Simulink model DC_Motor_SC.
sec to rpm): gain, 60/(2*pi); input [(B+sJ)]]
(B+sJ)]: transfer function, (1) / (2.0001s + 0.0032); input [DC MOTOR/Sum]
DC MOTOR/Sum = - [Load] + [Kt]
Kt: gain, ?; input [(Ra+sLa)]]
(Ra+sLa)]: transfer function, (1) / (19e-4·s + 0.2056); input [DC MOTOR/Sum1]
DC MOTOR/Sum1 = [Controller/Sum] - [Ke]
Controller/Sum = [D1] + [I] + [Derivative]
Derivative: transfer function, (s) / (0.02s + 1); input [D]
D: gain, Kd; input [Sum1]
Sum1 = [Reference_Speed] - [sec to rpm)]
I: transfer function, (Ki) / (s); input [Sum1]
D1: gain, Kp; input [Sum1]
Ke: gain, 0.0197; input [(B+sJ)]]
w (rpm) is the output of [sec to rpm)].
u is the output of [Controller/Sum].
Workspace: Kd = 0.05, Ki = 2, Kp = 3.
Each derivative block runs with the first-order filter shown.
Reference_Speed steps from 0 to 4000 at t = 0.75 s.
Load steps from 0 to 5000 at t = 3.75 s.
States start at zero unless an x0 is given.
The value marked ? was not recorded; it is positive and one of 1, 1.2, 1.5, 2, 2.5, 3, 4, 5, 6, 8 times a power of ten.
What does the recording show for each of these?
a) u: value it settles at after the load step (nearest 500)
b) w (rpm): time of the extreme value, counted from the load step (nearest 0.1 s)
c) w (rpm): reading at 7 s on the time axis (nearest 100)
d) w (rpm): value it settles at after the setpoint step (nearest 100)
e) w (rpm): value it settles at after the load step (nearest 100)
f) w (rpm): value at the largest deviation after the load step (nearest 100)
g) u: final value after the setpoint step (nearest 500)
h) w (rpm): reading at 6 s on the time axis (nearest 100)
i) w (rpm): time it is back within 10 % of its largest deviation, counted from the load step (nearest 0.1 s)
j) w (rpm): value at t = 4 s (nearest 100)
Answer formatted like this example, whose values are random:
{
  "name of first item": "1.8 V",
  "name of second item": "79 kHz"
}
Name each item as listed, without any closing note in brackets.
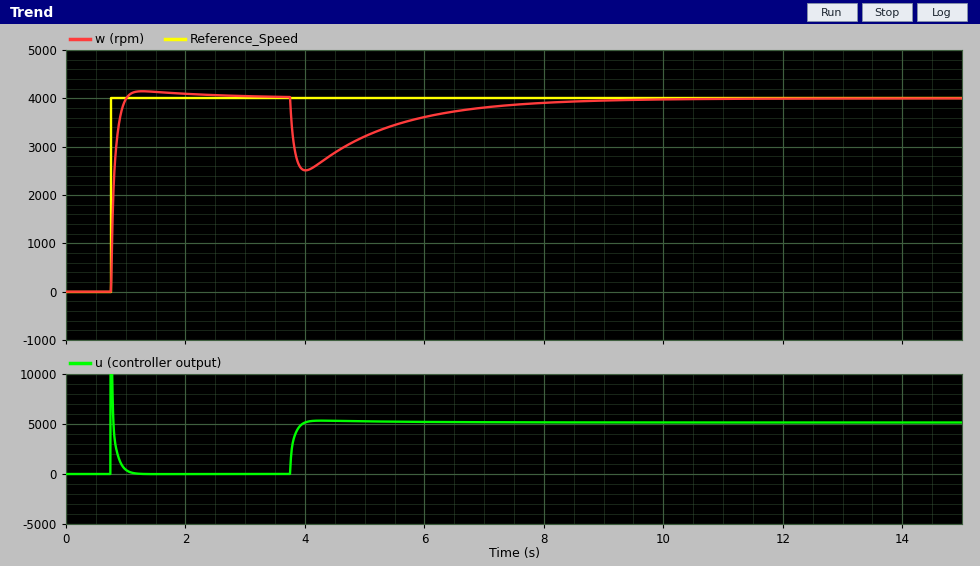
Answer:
{
  "u: value it settles at after the load step": "5000",
  "w (rpm): time of the extreme value, counted from the load step": "0.3 s",
  "w (rpm): reading at 7 s on the time axis": "3800",
  "w (rpm): value it settles at after the setpoint step": "4000",
  "w (rpm): value it settles at after the load step": "4000",
  "w (rpm): value at the largest deviation after the load step": "2500",
  "u: final value after the setpoint step": "0",
  "w (rpm): reading at 6 s on the time axis": "3600",
  "w (rpm): time it is back within 10 % of its largest deviation, counted from the load step": "3.6 s",
  "w (rpm): value at t = 4 s": "2500"
}
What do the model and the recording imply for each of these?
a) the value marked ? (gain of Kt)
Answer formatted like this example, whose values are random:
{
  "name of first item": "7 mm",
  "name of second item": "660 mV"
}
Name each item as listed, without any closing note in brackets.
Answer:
{
  "the value marked ?": "0.2"
}
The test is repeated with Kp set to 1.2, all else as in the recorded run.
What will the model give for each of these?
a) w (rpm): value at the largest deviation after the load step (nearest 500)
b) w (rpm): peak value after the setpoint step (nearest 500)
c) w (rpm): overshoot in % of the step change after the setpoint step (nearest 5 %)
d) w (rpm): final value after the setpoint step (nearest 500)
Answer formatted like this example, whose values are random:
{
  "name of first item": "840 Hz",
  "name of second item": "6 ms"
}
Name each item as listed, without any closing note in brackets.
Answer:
{
  "w (rpm): value at the largest deviation after the load step": "1000",
  "w (rpm): peak value after the setpoint step": "4500",
  "w (rpm): overshoot in % of the step change after the setpoint step": "15 %",
  "w (rpm): final value after the setpoint step": "4000"
}
